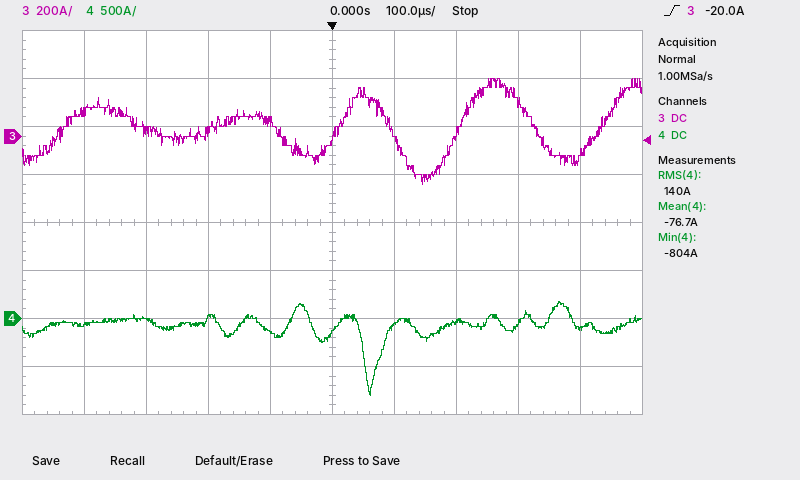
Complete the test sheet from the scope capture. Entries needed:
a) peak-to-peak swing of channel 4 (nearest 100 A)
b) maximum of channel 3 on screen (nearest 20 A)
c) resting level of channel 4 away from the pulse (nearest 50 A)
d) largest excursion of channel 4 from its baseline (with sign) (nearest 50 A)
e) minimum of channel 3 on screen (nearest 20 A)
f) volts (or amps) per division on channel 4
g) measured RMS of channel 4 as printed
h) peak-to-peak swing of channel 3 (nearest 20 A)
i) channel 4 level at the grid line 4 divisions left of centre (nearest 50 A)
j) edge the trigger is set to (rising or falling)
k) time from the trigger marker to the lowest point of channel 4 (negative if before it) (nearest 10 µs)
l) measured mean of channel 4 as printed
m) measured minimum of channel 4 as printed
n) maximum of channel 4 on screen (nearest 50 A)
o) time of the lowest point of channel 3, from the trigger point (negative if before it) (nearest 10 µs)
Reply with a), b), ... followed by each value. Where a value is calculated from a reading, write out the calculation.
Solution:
a) 1.00 kA
b) 240 A
c) -50 A
d) -750 A
e) -200 A
f) 500 A
g) 140 A
h) 240 A − (-200 A) = 440 A
i) -50 A
j) rising
k) +60 µs
l) -76.7 A
m) -804 A
n) 200 A
o) +150 µs
